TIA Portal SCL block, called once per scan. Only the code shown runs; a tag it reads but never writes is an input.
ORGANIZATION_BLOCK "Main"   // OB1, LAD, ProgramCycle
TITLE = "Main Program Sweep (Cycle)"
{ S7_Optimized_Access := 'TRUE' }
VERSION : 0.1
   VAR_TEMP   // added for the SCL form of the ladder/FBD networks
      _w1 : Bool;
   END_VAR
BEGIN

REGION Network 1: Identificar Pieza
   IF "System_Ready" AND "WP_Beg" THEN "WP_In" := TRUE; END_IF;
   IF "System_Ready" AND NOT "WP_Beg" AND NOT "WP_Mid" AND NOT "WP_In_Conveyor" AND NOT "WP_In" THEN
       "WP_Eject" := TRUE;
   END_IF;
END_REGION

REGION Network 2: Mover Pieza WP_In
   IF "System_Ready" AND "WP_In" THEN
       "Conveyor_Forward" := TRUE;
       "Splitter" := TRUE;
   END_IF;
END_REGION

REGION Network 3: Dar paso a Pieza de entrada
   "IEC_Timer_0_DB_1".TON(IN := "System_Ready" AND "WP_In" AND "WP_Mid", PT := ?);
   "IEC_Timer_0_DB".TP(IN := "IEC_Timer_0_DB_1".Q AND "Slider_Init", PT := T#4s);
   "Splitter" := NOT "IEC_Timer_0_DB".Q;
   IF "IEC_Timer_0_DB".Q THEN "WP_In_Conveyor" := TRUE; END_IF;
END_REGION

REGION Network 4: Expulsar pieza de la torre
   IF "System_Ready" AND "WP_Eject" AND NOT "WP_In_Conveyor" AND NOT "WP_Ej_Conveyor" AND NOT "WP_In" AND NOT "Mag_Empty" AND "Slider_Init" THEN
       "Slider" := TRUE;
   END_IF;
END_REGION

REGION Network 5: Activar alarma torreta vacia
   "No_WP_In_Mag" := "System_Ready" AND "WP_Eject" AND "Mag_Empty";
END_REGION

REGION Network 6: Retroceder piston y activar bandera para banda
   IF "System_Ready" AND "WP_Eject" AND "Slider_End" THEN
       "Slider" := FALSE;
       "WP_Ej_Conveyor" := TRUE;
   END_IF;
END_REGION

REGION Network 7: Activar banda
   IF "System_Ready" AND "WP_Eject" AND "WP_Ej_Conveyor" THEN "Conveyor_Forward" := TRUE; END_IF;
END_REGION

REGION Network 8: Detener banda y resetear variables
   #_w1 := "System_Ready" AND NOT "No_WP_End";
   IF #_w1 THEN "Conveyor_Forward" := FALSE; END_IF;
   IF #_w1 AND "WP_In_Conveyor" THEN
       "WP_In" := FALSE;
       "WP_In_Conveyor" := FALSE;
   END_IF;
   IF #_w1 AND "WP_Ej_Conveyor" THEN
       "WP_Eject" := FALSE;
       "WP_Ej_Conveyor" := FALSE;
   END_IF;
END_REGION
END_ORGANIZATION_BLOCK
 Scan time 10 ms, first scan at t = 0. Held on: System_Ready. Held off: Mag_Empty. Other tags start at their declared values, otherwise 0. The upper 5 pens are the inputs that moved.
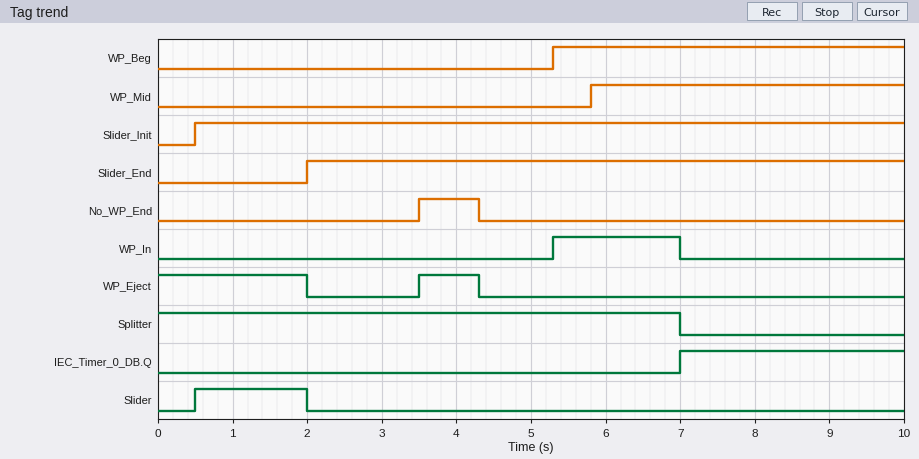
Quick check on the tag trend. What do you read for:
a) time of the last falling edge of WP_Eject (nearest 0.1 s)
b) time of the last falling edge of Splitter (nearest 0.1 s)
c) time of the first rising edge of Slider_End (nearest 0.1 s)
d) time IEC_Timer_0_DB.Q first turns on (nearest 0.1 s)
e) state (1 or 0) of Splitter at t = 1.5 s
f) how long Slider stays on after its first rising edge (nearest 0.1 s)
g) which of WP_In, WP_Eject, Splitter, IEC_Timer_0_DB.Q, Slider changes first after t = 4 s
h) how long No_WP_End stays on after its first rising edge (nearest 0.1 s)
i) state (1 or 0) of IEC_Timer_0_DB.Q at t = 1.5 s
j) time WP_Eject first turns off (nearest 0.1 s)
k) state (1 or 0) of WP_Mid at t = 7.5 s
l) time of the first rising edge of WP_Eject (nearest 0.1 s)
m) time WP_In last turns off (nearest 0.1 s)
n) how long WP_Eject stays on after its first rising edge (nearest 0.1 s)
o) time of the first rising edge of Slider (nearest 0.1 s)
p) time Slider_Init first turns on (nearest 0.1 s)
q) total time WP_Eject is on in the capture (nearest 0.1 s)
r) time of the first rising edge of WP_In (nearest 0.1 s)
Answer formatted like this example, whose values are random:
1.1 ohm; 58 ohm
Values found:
4.3 s; 7.0 s; 2.0 s; 7.0 s; 1; 1.5 s; WP_Eject; 0.8 s; 0; 2.0 s; 1; 3.5 s; 7.0 s; 0.8 s; 0.5 s; 0.5 s; 2.8 s; 5.3 s
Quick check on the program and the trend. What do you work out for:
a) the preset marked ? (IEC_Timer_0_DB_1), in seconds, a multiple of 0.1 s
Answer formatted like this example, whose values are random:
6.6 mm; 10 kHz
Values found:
1.2 s
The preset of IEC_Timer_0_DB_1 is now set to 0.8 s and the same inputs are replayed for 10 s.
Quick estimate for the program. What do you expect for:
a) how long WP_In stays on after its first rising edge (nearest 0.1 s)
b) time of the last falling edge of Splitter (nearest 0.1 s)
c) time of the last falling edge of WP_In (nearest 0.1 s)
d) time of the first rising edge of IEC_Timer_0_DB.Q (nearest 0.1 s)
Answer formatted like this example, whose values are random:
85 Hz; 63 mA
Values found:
1.3 s; 6.6 s; 6.6 s; 6.6 s
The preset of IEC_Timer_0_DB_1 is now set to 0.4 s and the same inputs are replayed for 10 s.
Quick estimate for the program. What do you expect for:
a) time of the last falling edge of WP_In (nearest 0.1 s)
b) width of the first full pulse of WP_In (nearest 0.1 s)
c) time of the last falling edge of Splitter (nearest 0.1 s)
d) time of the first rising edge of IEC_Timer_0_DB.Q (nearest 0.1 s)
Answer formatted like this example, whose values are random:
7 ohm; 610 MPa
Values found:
6.2 s; 0.9 s; 6.2 s; 6.2 s
